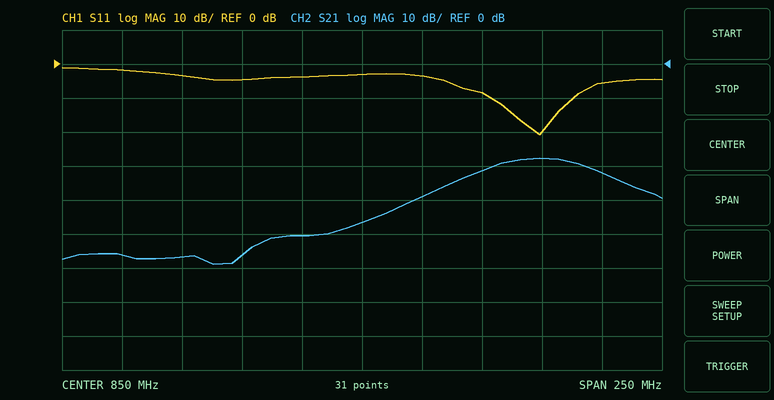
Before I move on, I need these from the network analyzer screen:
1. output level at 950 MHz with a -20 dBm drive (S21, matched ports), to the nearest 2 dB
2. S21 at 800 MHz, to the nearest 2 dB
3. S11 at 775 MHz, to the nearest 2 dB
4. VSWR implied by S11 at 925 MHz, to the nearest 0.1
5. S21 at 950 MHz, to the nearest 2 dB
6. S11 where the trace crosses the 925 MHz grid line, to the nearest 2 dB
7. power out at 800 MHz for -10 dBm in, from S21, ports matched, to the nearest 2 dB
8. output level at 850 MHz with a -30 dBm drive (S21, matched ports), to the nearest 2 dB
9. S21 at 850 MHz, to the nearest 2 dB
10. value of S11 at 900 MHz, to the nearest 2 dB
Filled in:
-52 dBm
-56 dB
-4 dB
1.2
-32 dB
-20 dB
-66 dBm
-76 dBm
-46 dB
-8 dB
